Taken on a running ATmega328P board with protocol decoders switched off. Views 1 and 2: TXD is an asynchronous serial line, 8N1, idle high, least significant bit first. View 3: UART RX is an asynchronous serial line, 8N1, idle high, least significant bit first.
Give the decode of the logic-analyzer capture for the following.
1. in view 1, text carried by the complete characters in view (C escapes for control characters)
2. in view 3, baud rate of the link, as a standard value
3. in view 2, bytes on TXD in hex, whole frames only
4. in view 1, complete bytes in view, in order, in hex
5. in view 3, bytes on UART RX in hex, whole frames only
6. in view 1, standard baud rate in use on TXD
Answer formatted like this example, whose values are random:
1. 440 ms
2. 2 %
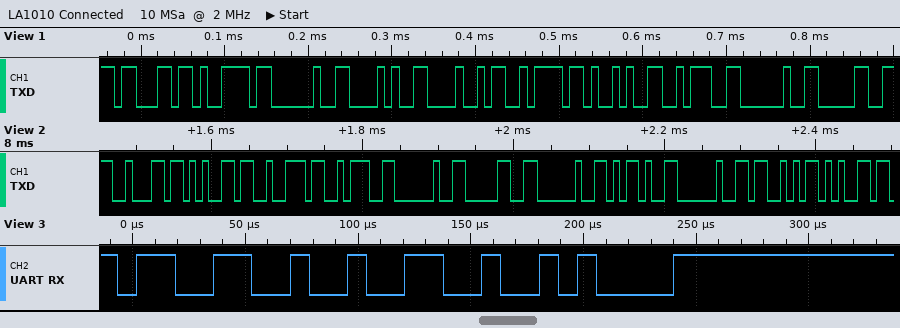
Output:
1. "cy (Hz): 0"
2. 115200 baud
3. 62 65 72 3A 20 30 20 2D 20 53 65
4. 0x63 0x79 0x20 0x28 0x48 0x7A 0x29 0x3A 0x20 0x30
5. 0x33 0x32 0x0A
6. 115200 baud
